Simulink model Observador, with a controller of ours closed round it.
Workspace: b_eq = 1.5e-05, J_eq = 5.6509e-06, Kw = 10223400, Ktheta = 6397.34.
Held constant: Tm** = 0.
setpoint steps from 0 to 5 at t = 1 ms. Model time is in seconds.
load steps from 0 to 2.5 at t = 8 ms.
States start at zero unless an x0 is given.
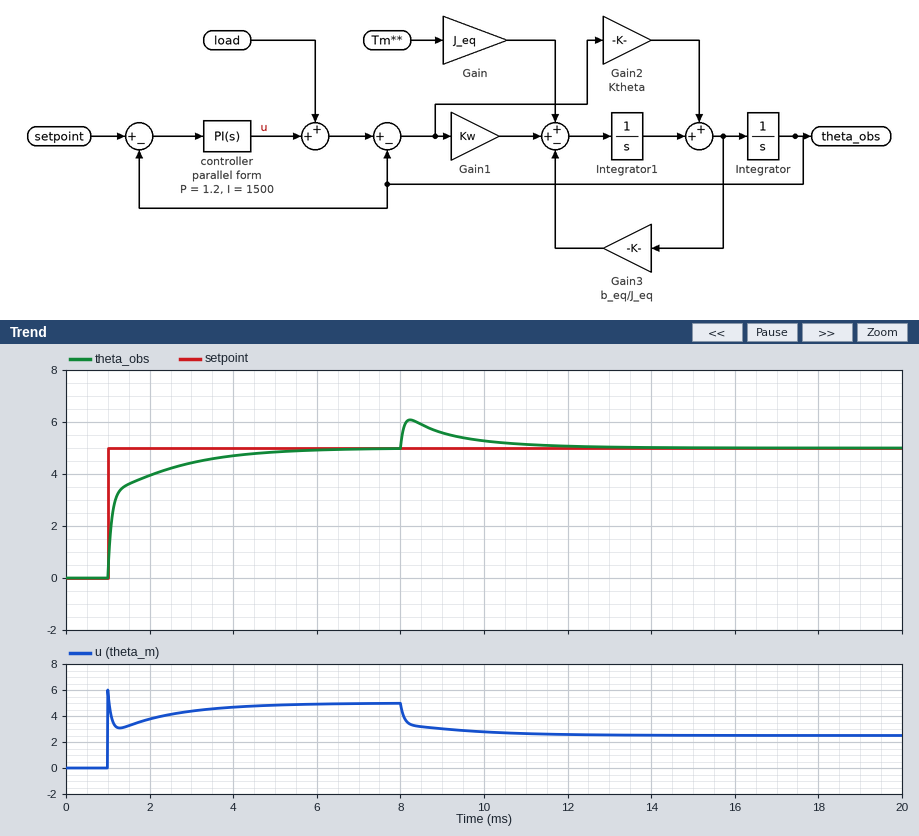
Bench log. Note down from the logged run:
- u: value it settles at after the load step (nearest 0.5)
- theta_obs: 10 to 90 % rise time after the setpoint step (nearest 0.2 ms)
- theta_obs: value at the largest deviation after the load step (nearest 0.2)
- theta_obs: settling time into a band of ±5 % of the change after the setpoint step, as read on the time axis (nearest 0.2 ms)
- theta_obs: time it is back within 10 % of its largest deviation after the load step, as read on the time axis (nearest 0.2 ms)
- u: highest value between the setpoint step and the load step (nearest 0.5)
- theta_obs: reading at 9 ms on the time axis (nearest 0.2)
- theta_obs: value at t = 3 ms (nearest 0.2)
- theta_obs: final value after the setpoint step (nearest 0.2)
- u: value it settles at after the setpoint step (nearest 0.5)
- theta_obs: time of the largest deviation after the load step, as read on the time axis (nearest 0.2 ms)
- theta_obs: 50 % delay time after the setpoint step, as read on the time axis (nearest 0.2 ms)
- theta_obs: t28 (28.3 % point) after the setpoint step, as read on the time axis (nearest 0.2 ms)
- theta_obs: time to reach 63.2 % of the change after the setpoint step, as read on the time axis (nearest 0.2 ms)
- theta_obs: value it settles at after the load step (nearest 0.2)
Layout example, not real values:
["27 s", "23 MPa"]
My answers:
["2.5", "2.2 ms", "6.0", "4.2 ms", "11.4 ms", "6.0", "5.6", "4.4", "5.0", "5.0", "8.2 ms", "1.2 ms", "1.0 ms", "1.2 ms", "5.0"]
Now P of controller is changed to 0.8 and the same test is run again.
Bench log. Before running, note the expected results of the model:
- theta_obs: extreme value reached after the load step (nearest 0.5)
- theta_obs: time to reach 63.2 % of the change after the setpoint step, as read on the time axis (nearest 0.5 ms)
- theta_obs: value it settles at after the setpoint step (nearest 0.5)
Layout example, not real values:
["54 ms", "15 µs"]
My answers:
["6.5", "1.5 ms", "5.0"]
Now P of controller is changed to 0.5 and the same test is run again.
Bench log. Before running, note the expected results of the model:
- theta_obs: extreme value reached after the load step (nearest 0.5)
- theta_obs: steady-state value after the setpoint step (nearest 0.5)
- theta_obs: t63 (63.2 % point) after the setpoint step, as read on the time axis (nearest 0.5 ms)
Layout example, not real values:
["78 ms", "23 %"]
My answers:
["6.5", "5.0", "1.5 ms"]
